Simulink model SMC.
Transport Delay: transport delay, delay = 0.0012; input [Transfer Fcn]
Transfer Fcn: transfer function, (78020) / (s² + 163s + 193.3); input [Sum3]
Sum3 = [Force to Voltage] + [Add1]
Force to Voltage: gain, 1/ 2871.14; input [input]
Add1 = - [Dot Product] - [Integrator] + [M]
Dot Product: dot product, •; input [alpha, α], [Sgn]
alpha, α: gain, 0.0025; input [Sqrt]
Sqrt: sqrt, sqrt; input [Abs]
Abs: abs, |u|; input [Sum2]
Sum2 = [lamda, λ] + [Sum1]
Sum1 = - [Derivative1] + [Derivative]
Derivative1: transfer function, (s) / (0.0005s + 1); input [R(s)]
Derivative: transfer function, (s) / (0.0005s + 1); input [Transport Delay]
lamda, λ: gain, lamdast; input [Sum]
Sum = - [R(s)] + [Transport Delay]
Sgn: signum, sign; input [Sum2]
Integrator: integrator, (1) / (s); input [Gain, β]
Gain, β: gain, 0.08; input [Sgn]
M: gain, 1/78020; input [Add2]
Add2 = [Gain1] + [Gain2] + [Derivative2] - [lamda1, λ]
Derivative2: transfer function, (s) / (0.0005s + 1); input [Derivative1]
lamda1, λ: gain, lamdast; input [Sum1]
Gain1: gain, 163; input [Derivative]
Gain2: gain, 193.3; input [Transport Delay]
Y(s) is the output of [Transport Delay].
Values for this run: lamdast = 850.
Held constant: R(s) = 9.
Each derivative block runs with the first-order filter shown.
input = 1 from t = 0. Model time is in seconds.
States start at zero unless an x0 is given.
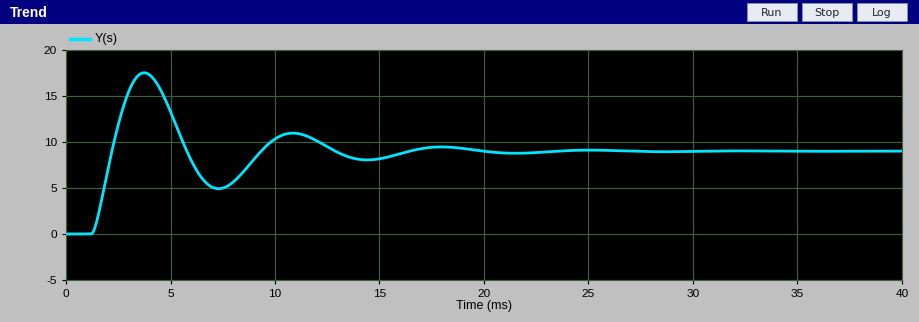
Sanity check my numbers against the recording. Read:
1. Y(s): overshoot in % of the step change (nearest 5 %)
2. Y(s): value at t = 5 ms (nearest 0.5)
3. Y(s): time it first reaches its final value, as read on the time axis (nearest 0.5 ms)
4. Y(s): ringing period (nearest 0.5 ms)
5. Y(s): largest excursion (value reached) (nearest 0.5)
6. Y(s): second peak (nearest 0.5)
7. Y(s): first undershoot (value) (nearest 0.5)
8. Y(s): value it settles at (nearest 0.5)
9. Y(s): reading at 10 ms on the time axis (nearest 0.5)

95 %
13.5
2.0 ms
7.0 ms
17.5
11.0
5.0
9.0
10.5
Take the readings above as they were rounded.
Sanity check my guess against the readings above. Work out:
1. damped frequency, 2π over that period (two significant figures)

0.90 rad/ms
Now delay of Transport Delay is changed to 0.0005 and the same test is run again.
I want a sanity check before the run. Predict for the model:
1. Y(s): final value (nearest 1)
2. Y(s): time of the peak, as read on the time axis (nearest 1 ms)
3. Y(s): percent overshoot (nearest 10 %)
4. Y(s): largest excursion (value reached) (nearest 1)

9
3 ms
50 %
14
